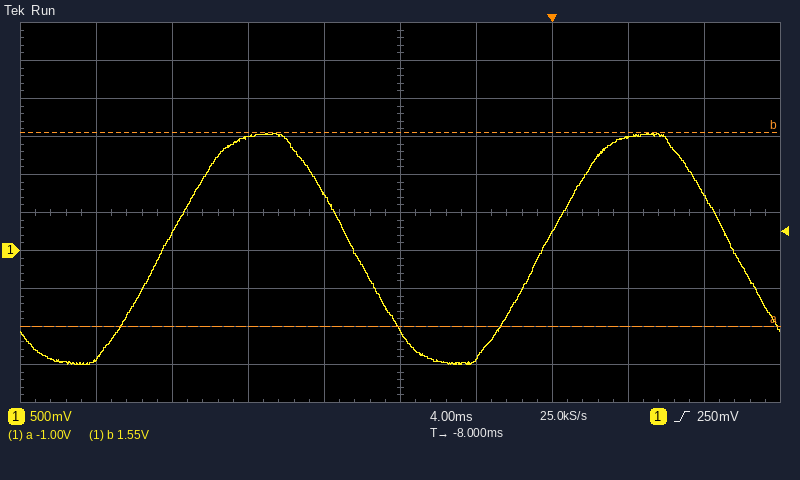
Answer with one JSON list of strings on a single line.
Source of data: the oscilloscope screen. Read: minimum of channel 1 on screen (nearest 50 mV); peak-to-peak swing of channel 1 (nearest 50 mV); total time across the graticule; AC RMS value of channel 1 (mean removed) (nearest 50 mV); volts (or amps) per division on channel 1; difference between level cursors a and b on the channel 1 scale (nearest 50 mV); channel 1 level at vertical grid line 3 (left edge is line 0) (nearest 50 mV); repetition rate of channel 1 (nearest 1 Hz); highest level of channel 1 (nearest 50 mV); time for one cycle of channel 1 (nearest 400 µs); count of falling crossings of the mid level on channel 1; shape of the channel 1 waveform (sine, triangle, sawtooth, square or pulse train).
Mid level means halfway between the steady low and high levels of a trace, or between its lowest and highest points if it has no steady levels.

["-1.50 V", "3.05 V", "40 ms", "1.10 V", "500 mV", "2.55 V", "1.50 V", "50 Hz", "1.55 V", "20.0 ms", "2", "sine"]
